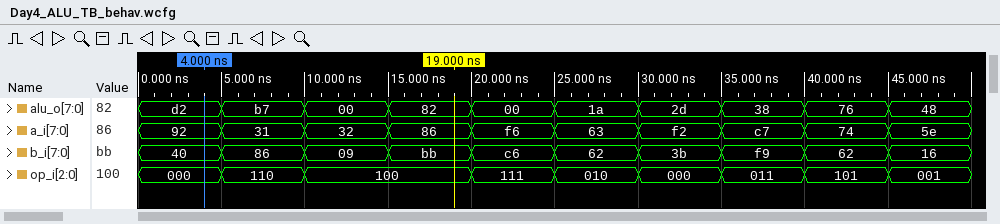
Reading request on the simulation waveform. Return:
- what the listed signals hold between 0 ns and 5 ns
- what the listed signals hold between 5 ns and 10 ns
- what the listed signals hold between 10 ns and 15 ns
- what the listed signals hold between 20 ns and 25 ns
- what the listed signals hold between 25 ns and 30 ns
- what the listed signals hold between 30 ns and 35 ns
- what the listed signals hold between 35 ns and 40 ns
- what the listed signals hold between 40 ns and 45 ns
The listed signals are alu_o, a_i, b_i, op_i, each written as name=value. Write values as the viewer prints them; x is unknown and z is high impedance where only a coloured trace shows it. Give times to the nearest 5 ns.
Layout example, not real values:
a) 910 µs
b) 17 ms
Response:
a) alu_o=d2, a_i=92, b_i=40, op_i=000
b) alu_o=b7, a_i=31, b_i=86, op_i=110
c) alu_o=00, a_i=32, b_i=09, op_i=100
d) alu_o=00, a_i=f6, b_i=c6, op_i=111
e) alu_o=1a, a_i=63, b_i=62, op_i=010
f) alu_o=2d, a_i=f2, b_i=3b, op_i=000
g) alu_o=38, a_i=c7, b_i=f9, op_i=011
h) alu_o=76, a_i=74, b_i=62, op_i=101
